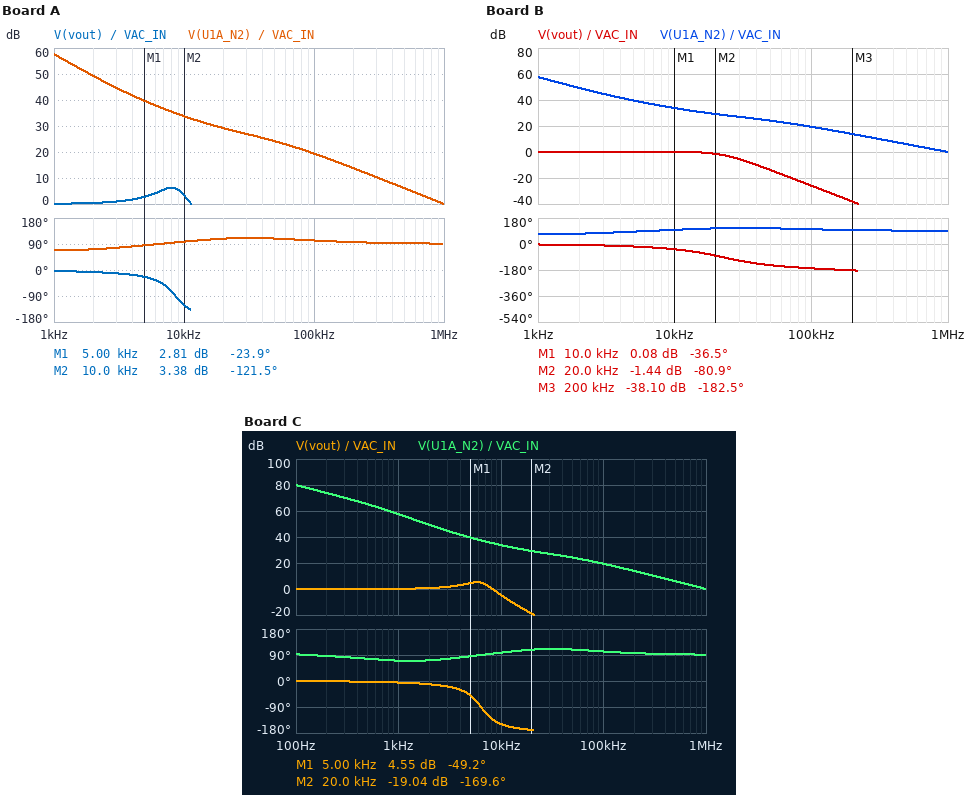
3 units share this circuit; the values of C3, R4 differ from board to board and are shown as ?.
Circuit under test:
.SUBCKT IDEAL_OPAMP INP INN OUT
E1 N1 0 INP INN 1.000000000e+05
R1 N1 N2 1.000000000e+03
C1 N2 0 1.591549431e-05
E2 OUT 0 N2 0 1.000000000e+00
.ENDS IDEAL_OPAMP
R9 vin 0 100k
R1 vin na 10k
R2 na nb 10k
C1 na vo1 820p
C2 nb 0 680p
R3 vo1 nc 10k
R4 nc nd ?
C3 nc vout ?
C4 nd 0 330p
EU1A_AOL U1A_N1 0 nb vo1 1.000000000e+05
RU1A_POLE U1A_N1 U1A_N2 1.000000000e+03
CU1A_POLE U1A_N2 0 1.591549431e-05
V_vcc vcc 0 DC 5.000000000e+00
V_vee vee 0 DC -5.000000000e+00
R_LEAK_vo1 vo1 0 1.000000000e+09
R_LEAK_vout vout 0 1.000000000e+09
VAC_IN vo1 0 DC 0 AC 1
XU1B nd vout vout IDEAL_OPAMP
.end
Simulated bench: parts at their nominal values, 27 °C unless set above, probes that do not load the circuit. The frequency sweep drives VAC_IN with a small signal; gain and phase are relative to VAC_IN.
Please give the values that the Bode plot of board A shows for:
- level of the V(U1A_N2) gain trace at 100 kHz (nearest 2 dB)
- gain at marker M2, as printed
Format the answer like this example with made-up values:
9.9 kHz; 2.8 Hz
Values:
20 dB; 3.38 dB
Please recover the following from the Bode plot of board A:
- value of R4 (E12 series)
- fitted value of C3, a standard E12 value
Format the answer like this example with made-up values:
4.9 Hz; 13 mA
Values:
18 kΩ; 5.6 nF
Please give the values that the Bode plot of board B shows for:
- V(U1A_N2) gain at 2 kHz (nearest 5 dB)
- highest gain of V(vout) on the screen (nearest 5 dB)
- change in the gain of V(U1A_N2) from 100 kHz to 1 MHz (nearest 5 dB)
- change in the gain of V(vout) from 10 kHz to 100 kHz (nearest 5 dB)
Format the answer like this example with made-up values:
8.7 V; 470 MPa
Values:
50 dB; 0 dB; -20 dB; -25 dB
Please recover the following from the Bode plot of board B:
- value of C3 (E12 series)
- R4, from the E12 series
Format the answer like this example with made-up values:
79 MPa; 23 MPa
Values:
820 pF; 18 kΩ
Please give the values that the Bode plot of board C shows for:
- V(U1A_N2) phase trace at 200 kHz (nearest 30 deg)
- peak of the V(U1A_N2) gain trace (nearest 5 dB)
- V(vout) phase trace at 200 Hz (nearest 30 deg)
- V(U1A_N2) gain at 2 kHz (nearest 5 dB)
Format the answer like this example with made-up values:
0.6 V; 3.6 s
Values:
90 deg; 80 dB; 0 deg; 50 dB
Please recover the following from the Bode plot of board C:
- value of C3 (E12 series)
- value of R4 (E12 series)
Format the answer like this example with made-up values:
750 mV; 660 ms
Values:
5.6 nF; 33 kΩ
